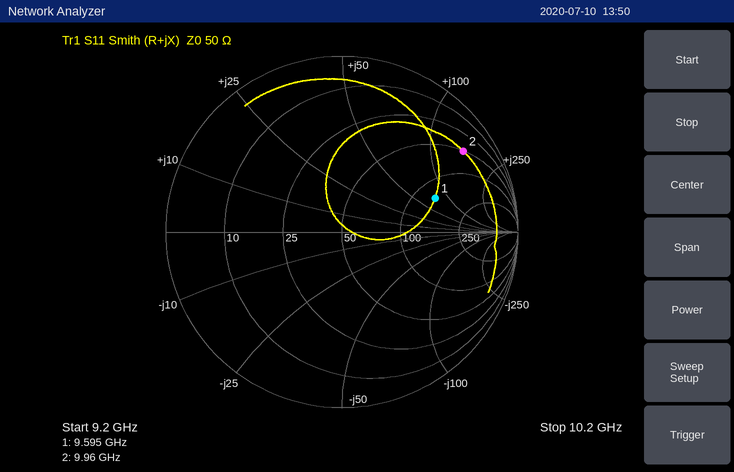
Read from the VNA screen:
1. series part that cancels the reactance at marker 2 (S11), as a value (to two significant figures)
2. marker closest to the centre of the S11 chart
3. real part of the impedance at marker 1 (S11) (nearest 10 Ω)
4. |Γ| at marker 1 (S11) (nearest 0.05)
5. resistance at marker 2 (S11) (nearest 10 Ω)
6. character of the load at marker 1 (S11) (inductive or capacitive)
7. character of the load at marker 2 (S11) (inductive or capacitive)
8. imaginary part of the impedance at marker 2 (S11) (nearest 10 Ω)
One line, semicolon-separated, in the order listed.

110 fF; marker 1; 130 Ω; 0.55; 50 Ω; inductive; inductive; +150 Ω
